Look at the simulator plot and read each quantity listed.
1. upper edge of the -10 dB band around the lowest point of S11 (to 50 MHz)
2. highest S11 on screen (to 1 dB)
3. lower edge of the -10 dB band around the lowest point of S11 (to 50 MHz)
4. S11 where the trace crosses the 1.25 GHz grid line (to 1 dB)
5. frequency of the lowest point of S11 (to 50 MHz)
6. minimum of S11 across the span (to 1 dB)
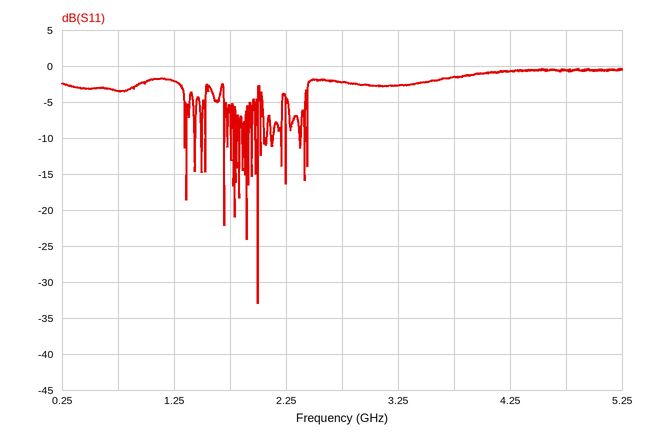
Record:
2.00 GHz
0 dB
2.00 GHz
-2 dB
2.00 GHz
-33 dB
